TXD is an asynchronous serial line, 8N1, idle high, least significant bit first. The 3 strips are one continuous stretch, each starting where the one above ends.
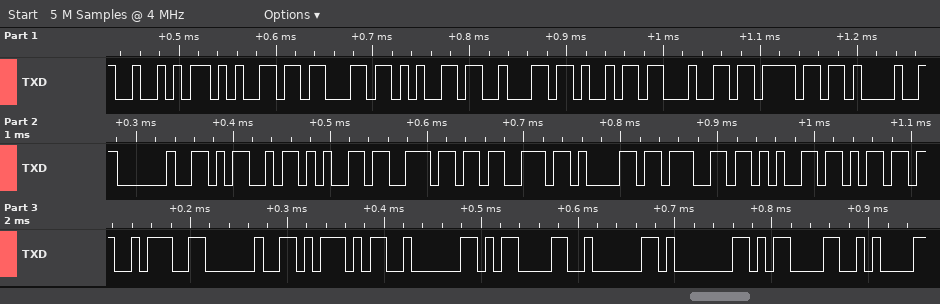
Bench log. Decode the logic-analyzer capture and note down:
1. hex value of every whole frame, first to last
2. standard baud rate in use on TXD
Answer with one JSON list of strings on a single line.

["52 65 63 65 62 69 64 6F 21 20 4D 65 6E 73 61 67 65 6D 3A 20 5D 02 0D 02 01 0D 0A", "115200 baud"]
